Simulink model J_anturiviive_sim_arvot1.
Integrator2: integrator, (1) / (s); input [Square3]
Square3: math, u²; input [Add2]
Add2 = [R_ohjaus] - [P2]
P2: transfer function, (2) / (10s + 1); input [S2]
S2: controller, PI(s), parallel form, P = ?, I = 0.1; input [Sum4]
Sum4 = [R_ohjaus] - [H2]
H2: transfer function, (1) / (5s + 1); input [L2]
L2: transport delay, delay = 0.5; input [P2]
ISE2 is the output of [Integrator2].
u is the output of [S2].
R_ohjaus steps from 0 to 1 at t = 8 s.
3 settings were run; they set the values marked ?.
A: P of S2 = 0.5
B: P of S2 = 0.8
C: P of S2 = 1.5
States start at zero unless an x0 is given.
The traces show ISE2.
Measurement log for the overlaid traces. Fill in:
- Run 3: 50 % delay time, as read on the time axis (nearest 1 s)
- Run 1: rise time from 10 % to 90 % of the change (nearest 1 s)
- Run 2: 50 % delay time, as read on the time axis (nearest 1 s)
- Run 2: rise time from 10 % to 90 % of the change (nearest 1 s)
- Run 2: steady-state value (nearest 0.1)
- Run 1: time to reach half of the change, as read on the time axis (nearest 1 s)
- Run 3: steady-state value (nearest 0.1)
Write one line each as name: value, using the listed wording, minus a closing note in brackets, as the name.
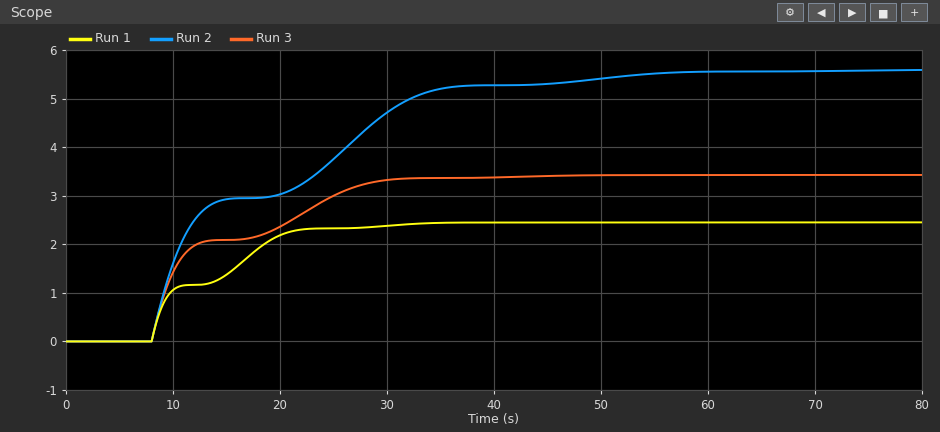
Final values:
Run 3: 50 % delay time, as read on the time axis: 11 s
Run 1: rise time from 10 % to 90 % of the change: 12 s
Run 2: 50 % delay time, as read on the time axis: 13 s
Run 2: rise time from 10 % to 90 % of the change: 24 s
Run 2: steady-state value: 5.6
Run 1: time to reach half of the change, as read on the time axis: 14 s
Run 3: steady-state value: 3.4
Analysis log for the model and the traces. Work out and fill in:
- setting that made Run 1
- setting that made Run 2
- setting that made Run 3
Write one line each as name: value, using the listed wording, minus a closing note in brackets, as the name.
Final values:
setting that made Run 1: C
setting that made Run 2: A
setting that made Run 3: B
